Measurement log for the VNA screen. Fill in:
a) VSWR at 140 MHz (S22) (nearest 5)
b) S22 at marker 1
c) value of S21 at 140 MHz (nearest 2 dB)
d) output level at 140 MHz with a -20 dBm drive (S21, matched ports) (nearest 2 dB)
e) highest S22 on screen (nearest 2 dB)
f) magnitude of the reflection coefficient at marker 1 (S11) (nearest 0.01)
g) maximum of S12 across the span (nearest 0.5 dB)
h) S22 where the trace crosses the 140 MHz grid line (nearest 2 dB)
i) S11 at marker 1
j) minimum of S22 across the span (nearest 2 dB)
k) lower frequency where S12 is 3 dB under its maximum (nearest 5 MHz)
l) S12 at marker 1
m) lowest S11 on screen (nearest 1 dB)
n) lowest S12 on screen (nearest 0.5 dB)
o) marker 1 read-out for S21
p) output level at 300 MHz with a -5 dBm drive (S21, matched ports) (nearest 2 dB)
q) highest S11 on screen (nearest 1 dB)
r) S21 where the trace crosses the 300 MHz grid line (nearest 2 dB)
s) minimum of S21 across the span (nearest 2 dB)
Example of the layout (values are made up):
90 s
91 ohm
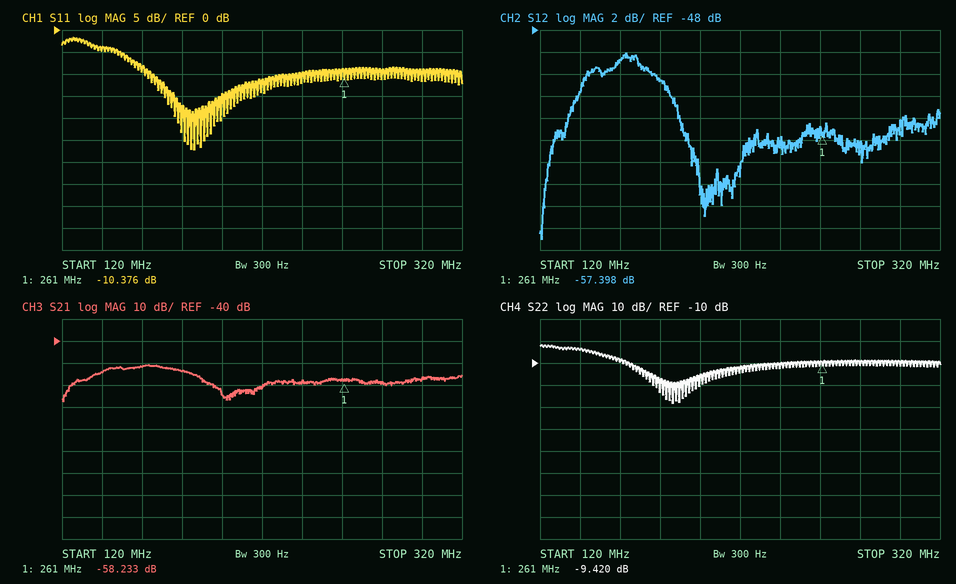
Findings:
5
-9.420 dB
-54 dB
-74 dBm
-2 dB
0.30
-50.0 dB
-4 dB
-10.376 dB
-28 dB
140 MHz
-57.398 dB
-27 dB
-67.0 dB
-58.233 dB
-62 dBm
-2 dB
-58 dB
-68 dB
